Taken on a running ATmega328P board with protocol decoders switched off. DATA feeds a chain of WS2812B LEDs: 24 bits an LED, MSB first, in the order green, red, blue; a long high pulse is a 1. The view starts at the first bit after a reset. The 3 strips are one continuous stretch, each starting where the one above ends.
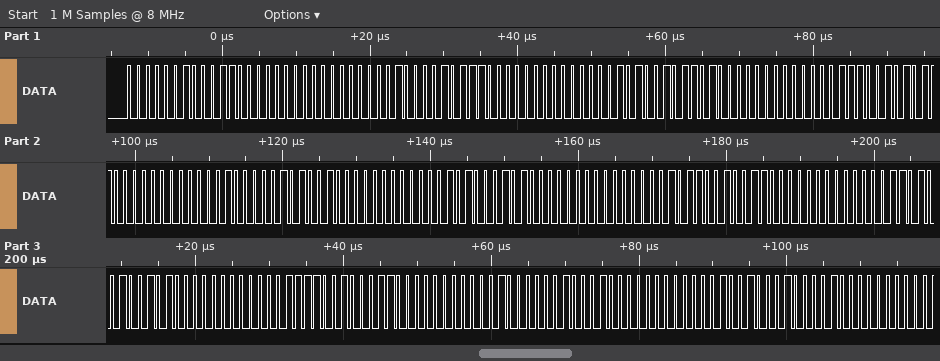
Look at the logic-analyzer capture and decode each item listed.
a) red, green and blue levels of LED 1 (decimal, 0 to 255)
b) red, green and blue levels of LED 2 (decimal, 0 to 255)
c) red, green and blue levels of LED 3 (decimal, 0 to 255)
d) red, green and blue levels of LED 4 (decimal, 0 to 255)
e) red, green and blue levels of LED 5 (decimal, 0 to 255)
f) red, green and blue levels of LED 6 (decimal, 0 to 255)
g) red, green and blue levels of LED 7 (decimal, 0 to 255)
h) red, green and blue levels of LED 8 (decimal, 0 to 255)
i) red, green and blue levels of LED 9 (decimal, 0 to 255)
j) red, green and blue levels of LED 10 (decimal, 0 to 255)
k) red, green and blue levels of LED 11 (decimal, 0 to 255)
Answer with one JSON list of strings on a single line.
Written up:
["48, 2, 0", "46, 4, 0", "45, 5, 0", "43, 7, 0", "41, 8, 0", "40, 10, 0", "38, 11, 0", "37, 13, 0", "35, 15, 0", "34, 16, 0", "33, 18, 0"]
